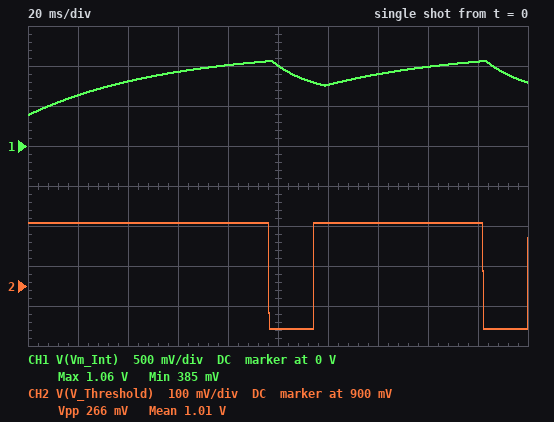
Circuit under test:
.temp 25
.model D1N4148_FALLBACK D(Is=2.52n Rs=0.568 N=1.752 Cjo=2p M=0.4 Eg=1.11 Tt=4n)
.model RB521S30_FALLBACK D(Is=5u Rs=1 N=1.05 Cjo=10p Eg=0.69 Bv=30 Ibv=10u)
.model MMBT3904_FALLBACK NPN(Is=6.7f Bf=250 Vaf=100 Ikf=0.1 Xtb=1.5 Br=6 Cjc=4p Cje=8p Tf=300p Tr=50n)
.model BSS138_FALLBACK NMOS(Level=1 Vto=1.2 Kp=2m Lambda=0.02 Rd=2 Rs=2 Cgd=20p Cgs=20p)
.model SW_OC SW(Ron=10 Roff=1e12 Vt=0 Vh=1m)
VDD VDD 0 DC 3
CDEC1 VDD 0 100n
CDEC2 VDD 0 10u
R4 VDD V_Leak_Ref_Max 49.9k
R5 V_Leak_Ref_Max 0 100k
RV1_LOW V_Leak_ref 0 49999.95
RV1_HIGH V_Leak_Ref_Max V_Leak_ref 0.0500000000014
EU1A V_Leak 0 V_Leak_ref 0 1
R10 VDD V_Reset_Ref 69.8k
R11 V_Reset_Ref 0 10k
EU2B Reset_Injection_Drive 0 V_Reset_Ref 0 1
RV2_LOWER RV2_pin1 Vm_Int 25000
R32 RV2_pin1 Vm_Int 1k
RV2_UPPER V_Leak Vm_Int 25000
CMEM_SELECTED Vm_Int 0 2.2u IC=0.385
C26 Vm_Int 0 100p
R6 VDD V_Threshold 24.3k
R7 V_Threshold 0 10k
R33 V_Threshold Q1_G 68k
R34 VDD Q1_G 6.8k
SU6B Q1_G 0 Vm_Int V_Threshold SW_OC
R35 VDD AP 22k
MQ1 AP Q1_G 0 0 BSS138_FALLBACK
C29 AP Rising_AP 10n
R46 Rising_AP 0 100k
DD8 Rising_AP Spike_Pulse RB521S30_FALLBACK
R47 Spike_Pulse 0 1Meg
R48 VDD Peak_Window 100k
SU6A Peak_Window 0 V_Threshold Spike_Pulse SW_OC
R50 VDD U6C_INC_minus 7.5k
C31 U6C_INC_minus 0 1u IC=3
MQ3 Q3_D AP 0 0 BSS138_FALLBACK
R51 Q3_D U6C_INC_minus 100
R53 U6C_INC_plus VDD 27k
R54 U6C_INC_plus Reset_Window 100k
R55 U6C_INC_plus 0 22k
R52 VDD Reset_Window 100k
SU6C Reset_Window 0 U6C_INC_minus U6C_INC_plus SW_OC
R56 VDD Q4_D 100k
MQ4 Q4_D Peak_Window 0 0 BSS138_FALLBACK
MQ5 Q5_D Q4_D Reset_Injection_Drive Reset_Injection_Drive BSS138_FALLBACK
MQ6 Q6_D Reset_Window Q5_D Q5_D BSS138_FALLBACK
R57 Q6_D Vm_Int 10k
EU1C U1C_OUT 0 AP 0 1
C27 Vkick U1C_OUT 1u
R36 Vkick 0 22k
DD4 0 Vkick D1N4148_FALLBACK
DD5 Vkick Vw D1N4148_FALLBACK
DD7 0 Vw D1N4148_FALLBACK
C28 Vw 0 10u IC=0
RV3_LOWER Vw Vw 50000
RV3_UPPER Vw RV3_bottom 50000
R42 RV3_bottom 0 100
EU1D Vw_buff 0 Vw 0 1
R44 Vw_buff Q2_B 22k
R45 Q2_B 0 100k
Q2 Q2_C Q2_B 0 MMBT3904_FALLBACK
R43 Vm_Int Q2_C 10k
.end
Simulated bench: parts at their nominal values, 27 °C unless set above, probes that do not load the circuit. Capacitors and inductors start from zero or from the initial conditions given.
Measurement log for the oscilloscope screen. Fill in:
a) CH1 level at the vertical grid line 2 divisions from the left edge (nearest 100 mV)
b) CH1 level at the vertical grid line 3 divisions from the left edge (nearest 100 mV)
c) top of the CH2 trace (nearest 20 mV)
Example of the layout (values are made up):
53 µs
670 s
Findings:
800 mV
900 mV
1.06 V
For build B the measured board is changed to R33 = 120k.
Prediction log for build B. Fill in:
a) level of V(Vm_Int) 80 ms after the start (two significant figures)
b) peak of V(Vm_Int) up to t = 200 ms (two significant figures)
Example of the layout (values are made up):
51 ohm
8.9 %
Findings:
900 mV
990 mV
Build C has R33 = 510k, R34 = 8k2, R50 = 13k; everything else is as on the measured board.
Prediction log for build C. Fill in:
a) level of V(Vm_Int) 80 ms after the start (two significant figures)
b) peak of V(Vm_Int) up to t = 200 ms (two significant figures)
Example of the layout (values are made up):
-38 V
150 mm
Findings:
860 mV
910 mV
